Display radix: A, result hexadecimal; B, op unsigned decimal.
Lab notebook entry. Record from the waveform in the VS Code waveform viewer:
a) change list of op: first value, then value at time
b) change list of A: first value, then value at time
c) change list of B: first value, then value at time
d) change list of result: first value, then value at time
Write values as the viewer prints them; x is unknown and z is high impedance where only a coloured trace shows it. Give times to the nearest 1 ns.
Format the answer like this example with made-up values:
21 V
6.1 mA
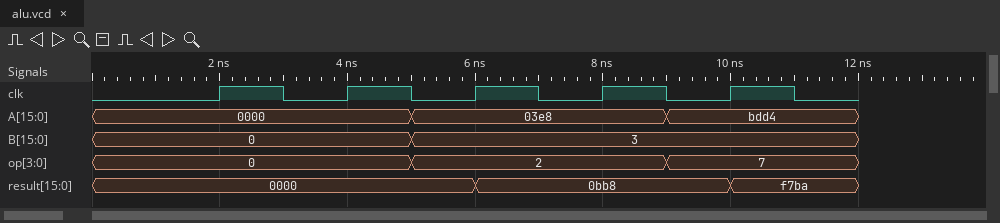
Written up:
0, 2 at 5 ns, 7 at 9 ns
0000, 03e8 at 5 ns, bdd4 at 9 ns
0, 3 at 5 ns
0000, 0bb8 at 6 ns, f7ba at 10 ns
